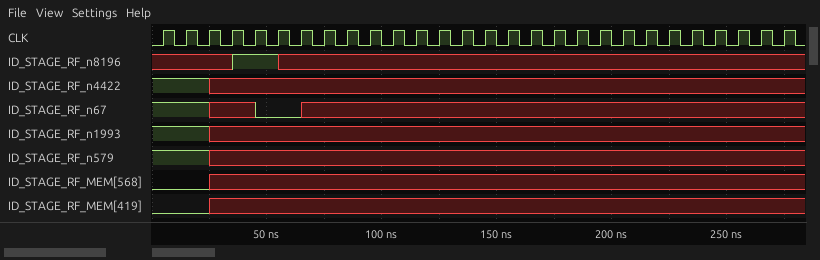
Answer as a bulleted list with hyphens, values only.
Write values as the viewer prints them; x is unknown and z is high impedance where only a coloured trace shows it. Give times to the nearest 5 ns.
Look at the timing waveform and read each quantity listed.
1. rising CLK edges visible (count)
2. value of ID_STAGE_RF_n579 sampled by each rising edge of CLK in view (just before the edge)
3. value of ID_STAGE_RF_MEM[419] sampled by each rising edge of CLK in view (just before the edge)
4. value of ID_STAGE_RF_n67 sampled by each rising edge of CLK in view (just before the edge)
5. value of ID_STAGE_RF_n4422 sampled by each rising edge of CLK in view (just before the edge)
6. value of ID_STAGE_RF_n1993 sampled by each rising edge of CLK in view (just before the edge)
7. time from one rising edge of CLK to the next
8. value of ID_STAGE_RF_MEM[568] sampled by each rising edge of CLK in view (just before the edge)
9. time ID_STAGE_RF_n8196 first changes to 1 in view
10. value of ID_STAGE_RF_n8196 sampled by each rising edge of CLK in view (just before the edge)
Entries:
- 28
- 1 1 1 x x x x x x x x x x x x x x x x x x x x x x x x x
- 0 0 0 x x x x x x x x x x x x x x x x x x x x x x x x x
- 1 1 1 x x 0 0 x x x x x x x x x x x x x x x x x x x x x
- 1 1 1 x x x x x x x x x x x x x x x x x x x x x x x x x
- 1 1 1 x x x x x x x x x x x x x x x x x x x x x x x x x
- 10 ns
- 0 0 0 x x x x x x x x x x x x x x x x x x x x x x x x x
- 35 ns
- x x x x 1 1 x x x x x x x x x x x x x x x x x x x x x x
